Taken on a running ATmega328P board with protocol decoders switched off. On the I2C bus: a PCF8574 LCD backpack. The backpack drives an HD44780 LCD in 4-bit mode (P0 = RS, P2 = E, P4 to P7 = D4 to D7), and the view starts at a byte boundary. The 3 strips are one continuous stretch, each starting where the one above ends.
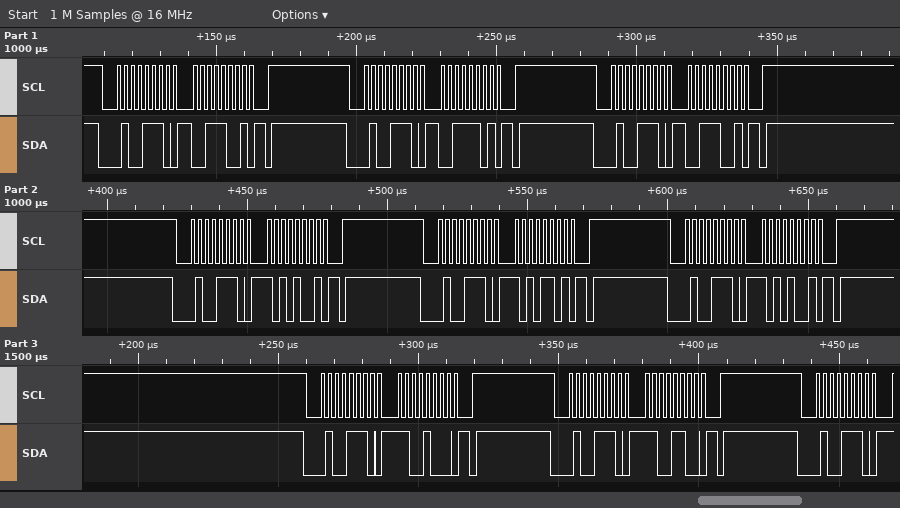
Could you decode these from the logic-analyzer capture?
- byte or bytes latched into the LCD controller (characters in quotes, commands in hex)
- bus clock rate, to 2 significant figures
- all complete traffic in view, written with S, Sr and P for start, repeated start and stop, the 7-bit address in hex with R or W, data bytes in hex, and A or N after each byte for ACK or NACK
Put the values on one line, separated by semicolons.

':'; 400 kHz; S 27W A 39 A P S 27W A 3D A P S 27W A 39 A P S 27W A A9 A P S 27W A AD A P S 27W A A9 A P S 27W A C8 A P S 27W A CC A P S 27W A
